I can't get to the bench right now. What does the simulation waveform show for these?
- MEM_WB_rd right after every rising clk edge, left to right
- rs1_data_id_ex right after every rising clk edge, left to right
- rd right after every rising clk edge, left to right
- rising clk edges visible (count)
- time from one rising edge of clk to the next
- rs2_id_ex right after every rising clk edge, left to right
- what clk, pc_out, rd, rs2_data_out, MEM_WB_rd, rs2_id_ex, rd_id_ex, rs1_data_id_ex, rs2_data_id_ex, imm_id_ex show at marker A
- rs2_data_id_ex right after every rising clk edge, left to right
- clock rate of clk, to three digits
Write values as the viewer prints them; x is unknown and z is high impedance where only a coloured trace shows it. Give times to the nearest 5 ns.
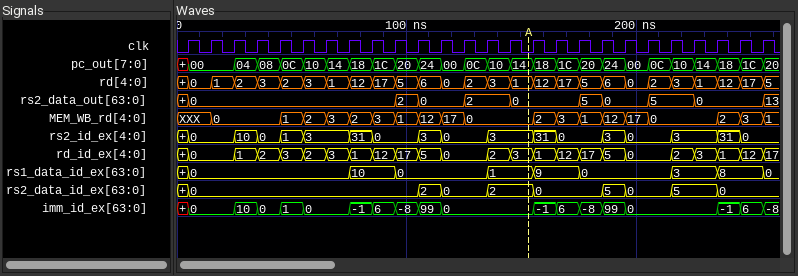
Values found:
XXX, 0, 0, 0, 1, 2, 3, 2, 3, 1, 12, 17, 0, 0, 0, 2, 3, 1, 12, 17, 0, 0, 0, 2, 3, 1
0, 0, 0, 0, 0, 0, 0, 10, 10, 0, 0, 0, 0, 1, 1, 9, 9, 0, 0, 0, 0, 3, 3, 8, 8, 0
0, 1, 2, 3, 2, 3, 1, 12, 17, 5, 6, 0, 2, 3, 1, 12, 17, 5, 6, 0, 2, 3, 1, 12, 17, 5
26
10 ns
0, 0, 10, 0, 1, 3, 3, 31, 0, 0, 3, 0, 0, 3, 3, 31, 0, 0, 3, 0, 0, 3, 3, 31, 0, 0
clk=0, pc_out=14, rd=1, rs2_data_out=0, MEM_WB_rd=0, rs2_id_ex=3, rd_id_ex=3, rs1_data_id_ex=1, rs2_data_id_ex=2, imm_id_ex=0
0, 0, 0, 0, 0, 0, 0, 0, 0, 0, 2, 0, 0, 2, 2, 0, 0, 0, 5, 0, 0, 5, 5, 0, 0, 0
100 MHz
